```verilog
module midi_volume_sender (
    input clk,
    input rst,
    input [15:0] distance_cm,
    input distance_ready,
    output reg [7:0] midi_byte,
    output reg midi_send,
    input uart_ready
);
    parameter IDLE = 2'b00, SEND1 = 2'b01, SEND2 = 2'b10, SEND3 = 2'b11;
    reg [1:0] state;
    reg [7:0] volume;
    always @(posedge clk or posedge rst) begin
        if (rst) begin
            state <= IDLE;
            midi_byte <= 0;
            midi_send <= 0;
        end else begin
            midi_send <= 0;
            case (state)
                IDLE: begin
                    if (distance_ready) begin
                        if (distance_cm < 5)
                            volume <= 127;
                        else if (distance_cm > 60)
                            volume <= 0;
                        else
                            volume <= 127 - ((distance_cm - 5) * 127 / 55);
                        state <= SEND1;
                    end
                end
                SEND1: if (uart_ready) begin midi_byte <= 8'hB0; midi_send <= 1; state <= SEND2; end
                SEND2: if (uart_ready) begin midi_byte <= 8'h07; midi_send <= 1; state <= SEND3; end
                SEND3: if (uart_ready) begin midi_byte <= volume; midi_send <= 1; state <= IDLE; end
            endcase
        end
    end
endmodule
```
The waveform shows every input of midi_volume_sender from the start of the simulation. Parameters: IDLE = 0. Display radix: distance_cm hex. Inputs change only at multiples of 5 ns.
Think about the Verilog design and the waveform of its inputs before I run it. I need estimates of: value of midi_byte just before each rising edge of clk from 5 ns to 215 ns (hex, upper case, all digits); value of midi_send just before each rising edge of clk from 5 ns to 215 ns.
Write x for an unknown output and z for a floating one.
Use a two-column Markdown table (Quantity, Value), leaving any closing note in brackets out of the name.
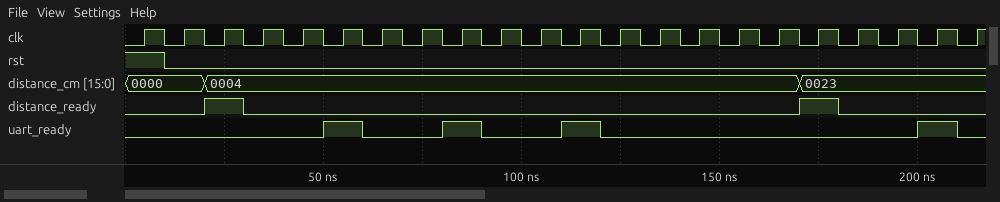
| Quantity | Value |
|---|---|
| value of midi_byte just before each rising edge of clk from 5 ns to 215 ns | 00, 00, 00, 00, 00, 00, B0, B0, B0, 07, 07, 07, 7F, 7F, 7F, 7F, 7F, 7F, 7F, 7F, 7F, B0 |
| value of midi_send just before each rising edge of clk from 5 ns to 215 ns | 0 0 0 0 0 0 1 0 0 1 0 0 1 0 0 0 0 0 0 0 0 1 |
